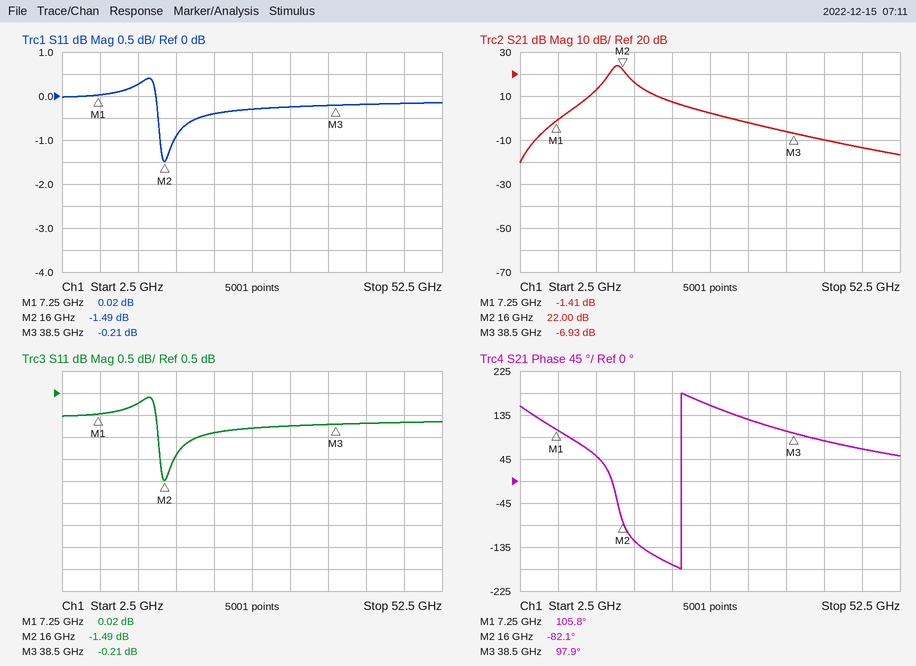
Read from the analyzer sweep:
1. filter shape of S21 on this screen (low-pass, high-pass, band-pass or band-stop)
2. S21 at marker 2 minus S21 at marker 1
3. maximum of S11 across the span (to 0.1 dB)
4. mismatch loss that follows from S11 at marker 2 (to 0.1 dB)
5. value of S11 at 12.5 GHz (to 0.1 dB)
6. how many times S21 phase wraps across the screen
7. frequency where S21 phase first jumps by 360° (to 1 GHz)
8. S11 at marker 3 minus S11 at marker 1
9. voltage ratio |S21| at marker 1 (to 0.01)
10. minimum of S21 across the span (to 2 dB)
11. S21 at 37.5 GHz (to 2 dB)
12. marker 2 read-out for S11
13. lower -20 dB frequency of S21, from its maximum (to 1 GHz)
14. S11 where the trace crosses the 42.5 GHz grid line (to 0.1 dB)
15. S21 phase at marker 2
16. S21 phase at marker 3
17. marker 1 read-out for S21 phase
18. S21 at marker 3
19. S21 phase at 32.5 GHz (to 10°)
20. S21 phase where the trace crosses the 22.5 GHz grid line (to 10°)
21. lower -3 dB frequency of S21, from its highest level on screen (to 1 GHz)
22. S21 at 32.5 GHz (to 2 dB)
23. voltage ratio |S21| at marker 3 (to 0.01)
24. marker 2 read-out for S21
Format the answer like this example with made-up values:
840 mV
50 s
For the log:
band-pass
23.41 dB
0.4 dB
5.4 dB
0.3 dB
1
24 GHz
-0.23 dB
0.85
-20 dB
-6 dB
-1.49 dB
9 GHz
-0.2 dB
-82.1°
97.9°
105.8°
-6.93 dB
130°
-170°
14 GHz
-2 dB
0.45
22.00 dB
